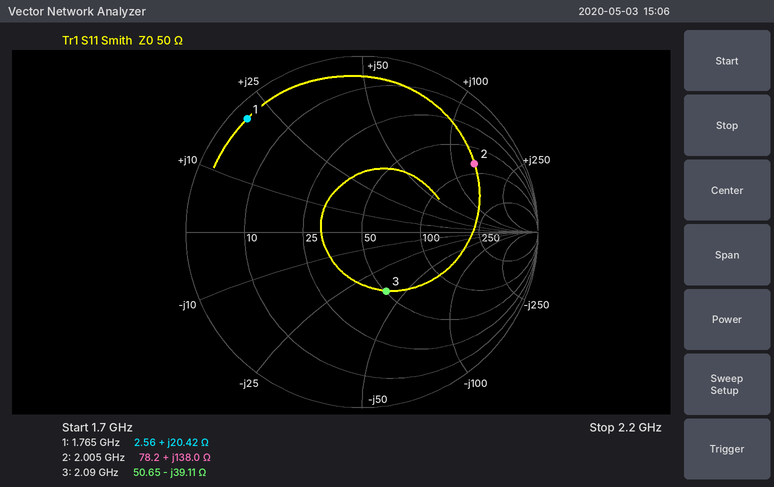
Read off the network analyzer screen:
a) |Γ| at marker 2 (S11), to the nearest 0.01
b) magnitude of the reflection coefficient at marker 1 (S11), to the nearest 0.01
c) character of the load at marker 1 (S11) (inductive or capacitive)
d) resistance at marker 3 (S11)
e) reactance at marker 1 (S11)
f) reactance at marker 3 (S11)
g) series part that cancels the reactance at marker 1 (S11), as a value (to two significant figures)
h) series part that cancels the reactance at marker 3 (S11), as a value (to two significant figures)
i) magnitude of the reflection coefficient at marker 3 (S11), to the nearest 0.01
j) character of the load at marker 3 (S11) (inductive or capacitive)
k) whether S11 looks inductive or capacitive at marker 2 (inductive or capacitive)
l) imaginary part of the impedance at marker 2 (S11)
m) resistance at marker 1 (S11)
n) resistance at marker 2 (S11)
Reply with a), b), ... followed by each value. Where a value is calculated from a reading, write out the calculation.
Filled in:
a) 0.75
b) 0.92
c) inductive
d) 50.65 Ω
e) +20.42 Ω
f) -39.11 Ω
g) C = 1/(2π × 1.765 GHz × 20.42 Ω) ≈ 4.4 pF
h) L = 39.11 Ω/(2π × 2.09 GHz) ≈ 3.0 nH
i) 0.36
j) capacitive
k) inductive
l) +138.0 Ω
m) 2.56 Ω
n) 78.2 Ω
